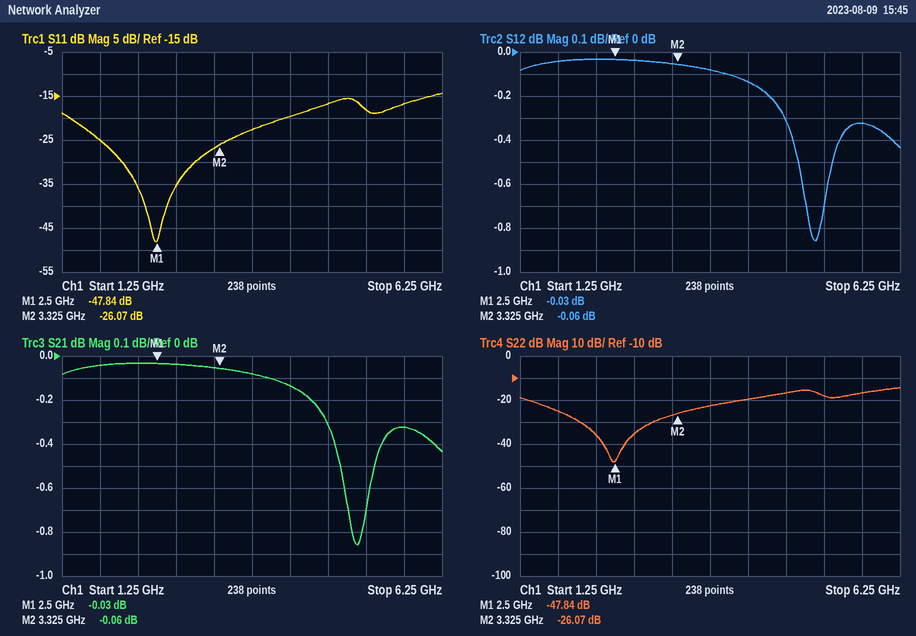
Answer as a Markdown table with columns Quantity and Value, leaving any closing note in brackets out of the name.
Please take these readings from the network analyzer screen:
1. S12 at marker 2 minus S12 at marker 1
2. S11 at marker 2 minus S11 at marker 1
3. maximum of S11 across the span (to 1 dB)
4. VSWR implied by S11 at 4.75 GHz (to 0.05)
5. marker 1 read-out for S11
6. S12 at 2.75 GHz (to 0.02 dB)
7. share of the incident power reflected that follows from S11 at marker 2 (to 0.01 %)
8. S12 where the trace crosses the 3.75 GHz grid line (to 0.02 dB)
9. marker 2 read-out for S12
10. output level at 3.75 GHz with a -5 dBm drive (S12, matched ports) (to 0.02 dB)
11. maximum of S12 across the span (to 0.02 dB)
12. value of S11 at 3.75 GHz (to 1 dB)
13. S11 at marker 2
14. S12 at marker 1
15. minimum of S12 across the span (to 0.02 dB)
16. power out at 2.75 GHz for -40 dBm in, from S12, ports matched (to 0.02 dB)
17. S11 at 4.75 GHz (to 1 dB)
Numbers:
| Quantity | Value |
|---|---|
| S12 at marker 2 minus S12 at marker 1 | -0.03 dB |
| S11 at marker 2 minus S11 at marker 1 | 21.77 dB |
| maximum of S11 across the span | -14 dB |
| VSWR implied by S11 at 4.75 GHz | 1.35 |
| marker 1 read-out for S11 | -47.84 dB |
| S12 at 2.75 GHz | -0.04 dB |
| share of the incident power reflected that follows from S11 at marker 2 | 0.25 % |
| S12 where the trace crosses the 3.75 GHz grid line | -0.08 dB |
| marker 2 read-out for S12 | -0.06 dB |
| output level at 3.75 GHz with a -5 dBm drive (S12, matched ports) | -5.08 dBm |
| maximum of S12 across the span | -0.04 dB |
| value of S11 at 3.75 GHz | -23 dB |
| S11 at marker 2 | -26.07 dB |
| S12 at marker 1 | -0.03 dB |
| minimum of S12 across the span | -0.86 dB |
| power out at 2.75 GHz for -40 dBm in, from S12, ports matched | -40.04 dBm |
| S11 at 4.75 GHz | -17 dB |
